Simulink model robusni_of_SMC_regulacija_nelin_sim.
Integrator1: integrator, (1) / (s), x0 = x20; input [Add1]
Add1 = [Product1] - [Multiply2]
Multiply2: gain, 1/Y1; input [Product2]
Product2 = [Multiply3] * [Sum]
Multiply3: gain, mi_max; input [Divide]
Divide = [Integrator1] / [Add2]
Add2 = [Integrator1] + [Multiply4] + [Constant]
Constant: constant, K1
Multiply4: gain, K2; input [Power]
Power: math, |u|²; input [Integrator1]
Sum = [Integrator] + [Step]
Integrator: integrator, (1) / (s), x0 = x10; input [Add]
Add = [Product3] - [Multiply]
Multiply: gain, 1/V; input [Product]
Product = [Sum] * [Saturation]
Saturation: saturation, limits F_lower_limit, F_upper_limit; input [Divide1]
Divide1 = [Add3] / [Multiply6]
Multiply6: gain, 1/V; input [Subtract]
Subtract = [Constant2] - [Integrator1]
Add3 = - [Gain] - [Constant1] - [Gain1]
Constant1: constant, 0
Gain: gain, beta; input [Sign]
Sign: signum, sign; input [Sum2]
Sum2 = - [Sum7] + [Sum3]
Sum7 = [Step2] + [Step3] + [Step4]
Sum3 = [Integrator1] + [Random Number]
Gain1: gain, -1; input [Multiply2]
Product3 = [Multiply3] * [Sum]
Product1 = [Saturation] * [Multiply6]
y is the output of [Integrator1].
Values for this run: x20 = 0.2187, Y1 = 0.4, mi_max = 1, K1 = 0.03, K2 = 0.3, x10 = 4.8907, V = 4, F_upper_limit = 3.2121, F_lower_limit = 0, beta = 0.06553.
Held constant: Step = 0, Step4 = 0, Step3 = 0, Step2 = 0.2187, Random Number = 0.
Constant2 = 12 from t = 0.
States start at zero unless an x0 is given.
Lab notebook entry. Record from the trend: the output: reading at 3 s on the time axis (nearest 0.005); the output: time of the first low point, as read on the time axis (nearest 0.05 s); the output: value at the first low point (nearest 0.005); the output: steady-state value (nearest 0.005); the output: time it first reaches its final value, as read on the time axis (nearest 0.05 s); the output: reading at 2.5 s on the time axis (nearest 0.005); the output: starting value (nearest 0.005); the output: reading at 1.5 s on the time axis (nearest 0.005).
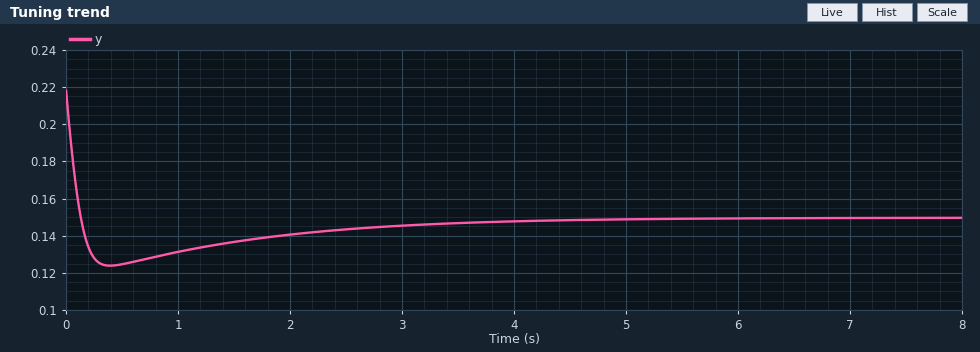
0.145
0.40 s
0.125
0.150
0.15 s
0.145
0.220
0.135
